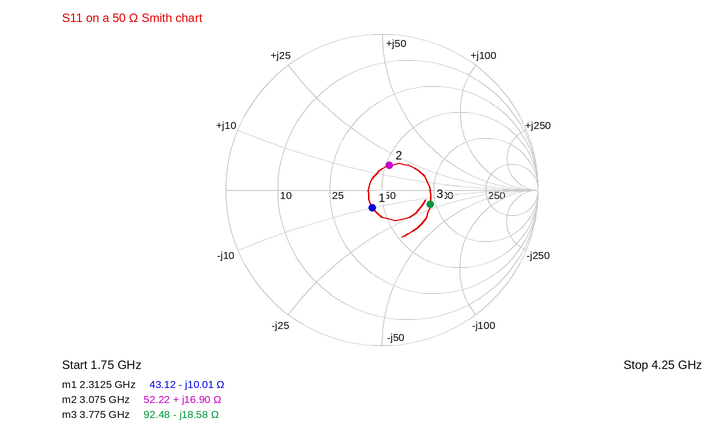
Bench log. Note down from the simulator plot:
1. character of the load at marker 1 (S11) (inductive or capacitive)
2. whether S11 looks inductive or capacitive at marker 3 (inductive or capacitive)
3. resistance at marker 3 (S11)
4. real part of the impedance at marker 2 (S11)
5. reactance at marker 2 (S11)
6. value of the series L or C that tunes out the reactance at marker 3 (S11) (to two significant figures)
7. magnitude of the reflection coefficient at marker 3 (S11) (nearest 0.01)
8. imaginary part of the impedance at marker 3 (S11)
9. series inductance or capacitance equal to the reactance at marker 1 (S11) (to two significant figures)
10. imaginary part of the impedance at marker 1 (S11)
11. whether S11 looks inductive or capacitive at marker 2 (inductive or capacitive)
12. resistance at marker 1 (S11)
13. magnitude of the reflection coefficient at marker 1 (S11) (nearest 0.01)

capacitive
capacitive
92.48 Ω
52.22 Ω
+16.90 Ω
780 pH
0.32
-18.58 Ω
6.9 pF
-10.01 Ω
inductive
43.12 Ω
0.13
